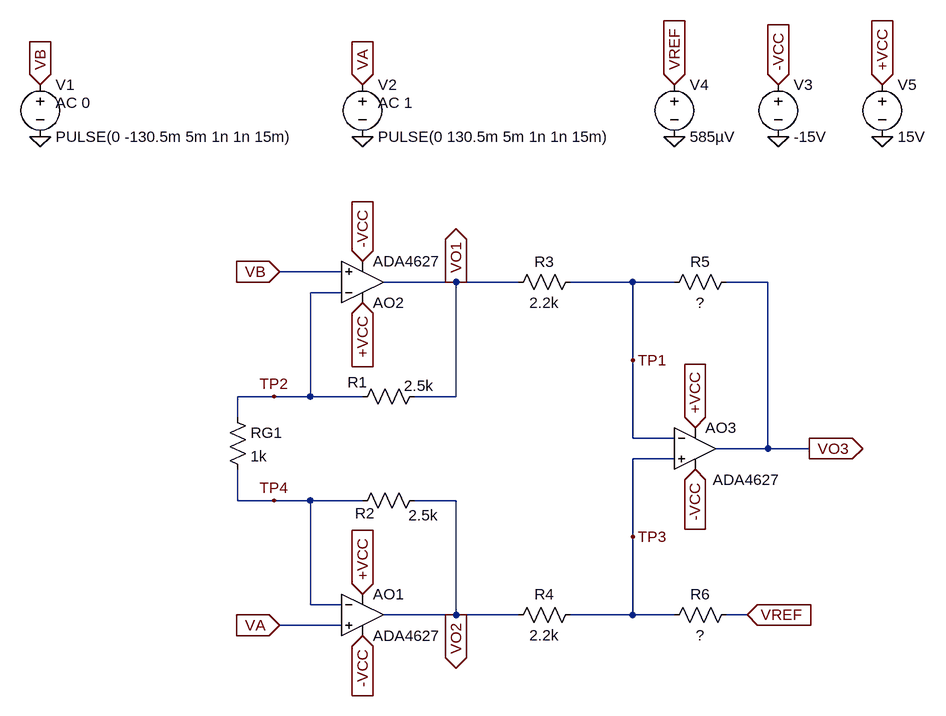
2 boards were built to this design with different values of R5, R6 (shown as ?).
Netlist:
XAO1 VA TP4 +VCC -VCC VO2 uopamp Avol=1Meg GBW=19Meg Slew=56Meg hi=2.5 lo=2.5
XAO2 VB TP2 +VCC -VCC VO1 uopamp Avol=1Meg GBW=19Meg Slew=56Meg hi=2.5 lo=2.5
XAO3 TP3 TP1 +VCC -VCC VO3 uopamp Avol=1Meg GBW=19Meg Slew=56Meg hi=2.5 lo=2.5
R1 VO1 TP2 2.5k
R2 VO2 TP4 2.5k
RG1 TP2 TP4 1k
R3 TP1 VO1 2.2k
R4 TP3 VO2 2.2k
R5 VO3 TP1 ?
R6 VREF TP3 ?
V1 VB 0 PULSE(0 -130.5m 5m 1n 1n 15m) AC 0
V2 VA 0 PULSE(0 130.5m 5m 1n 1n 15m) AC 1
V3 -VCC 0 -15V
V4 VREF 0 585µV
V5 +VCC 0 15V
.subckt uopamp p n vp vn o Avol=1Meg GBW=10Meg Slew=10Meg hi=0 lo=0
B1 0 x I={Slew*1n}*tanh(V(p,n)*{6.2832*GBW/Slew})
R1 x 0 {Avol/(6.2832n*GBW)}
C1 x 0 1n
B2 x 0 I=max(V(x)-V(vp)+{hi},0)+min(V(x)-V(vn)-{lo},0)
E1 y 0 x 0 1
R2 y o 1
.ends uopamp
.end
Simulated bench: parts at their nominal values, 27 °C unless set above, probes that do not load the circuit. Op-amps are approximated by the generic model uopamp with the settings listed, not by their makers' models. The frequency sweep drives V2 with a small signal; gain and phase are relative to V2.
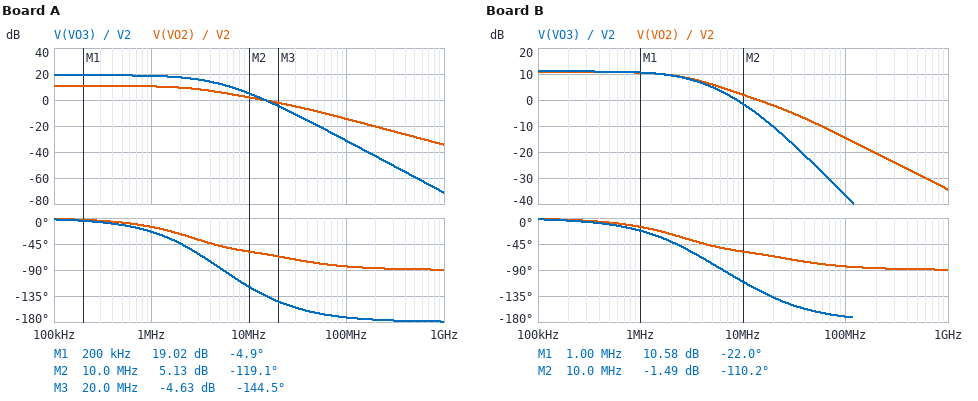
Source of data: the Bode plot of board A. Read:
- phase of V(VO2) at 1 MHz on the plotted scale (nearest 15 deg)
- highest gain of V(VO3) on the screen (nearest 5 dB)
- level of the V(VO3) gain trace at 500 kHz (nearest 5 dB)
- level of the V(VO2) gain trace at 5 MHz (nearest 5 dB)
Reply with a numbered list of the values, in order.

1. -15 deg
2. 20 dB
3. 20 dB
4. 5 dB
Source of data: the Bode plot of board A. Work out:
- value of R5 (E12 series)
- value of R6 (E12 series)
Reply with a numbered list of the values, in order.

1. 2.7 kΩ
2. 6.8 kΩ
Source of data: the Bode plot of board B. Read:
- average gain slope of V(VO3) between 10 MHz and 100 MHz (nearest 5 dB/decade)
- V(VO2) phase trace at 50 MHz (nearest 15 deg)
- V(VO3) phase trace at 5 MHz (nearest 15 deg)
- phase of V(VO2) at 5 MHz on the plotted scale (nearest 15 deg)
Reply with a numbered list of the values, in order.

1. -35 dB/decade
2. -75 deg
3. -75 deg
4. -45 deg
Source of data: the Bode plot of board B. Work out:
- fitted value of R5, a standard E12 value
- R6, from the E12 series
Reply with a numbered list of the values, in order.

1. 1.2 kΩ
2. 1.5 kΩ
